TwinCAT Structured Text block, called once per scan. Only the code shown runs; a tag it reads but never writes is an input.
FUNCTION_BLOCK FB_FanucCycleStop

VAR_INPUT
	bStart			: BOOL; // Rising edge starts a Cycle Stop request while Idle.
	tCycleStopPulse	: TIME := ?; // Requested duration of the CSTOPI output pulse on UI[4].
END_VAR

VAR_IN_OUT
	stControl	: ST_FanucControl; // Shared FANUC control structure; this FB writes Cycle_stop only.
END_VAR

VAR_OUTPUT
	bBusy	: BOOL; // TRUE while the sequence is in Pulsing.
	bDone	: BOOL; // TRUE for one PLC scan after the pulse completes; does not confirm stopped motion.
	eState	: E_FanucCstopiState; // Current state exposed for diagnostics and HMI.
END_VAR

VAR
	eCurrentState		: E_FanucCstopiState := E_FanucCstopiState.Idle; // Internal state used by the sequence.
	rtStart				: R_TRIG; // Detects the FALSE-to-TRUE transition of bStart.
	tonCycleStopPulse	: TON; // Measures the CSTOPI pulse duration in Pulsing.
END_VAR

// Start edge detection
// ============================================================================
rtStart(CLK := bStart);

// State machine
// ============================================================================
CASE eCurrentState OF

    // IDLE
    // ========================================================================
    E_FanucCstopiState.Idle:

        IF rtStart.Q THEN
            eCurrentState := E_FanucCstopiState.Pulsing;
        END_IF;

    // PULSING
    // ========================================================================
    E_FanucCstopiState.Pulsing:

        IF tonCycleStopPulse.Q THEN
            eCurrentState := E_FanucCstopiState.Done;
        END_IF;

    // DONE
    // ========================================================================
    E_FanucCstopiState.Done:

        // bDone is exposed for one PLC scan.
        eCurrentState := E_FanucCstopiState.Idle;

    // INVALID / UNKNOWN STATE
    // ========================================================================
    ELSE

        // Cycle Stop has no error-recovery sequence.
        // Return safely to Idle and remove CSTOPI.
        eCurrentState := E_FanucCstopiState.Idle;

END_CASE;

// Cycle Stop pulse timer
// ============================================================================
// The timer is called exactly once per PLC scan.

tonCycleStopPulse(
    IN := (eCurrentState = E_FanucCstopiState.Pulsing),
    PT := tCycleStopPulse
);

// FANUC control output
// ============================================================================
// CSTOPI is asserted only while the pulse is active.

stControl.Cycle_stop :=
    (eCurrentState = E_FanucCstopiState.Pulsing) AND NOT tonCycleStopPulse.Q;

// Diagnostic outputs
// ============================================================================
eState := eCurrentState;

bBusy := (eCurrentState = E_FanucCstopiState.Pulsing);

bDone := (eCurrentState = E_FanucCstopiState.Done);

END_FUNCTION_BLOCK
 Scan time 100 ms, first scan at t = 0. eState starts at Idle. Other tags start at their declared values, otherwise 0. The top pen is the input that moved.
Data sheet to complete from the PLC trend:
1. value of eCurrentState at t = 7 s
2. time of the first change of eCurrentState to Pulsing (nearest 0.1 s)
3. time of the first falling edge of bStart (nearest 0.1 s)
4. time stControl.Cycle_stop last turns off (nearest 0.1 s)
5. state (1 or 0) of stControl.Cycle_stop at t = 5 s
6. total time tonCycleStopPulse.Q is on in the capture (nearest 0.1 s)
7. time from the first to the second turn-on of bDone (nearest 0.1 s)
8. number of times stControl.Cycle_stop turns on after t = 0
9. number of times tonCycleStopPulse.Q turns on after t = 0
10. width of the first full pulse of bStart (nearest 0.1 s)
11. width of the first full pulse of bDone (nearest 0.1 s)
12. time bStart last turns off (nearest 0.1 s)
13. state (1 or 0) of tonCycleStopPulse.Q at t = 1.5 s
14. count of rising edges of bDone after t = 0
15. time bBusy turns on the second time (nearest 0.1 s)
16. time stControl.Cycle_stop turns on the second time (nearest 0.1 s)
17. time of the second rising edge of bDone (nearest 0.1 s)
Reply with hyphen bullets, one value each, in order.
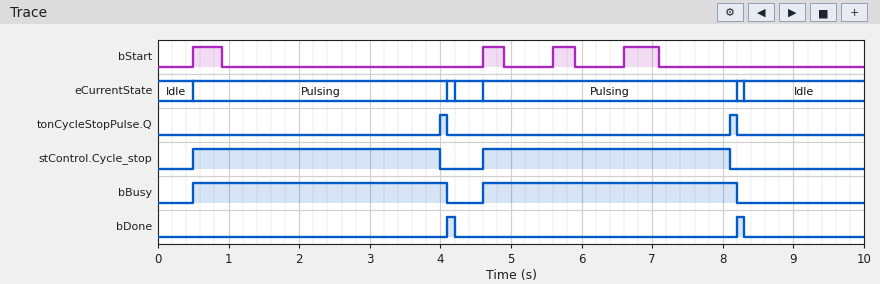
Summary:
- Pulsing
- 0.5 s
- 0.9 s
- 8.1 s
- 1
- 0.2 s
- 4.1 s
- 2
- 2
- 0.4 s
- 0.1 s
- 7.1 s
- 0
- 2
- 4.6 s
- 4.6 s
- 8.2 s
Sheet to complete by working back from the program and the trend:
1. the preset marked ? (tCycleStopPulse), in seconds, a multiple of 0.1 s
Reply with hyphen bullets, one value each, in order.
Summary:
- 3.5 s
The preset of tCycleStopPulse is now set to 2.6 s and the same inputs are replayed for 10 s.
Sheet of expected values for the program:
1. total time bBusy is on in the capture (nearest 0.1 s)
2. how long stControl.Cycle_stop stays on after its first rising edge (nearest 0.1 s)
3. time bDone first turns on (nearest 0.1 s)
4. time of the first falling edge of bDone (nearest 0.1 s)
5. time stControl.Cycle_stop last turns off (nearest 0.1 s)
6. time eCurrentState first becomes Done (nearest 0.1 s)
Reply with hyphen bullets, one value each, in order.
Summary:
- 5.4 s
- 2.6 s
- 3.2 s
- 3.3 s
- 7.2 s
- 3.2 s
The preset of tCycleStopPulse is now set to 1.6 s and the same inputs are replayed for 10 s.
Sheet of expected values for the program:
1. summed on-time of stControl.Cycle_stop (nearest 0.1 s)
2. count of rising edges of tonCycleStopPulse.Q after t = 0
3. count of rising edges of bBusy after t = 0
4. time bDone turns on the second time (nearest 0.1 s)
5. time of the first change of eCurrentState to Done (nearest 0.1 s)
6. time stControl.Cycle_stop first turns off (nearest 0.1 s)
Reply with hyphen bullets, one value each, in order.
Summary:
- 4.8 s
- 3
- 3
- 6.3 s
- 2.2 s
- 2.1 s
